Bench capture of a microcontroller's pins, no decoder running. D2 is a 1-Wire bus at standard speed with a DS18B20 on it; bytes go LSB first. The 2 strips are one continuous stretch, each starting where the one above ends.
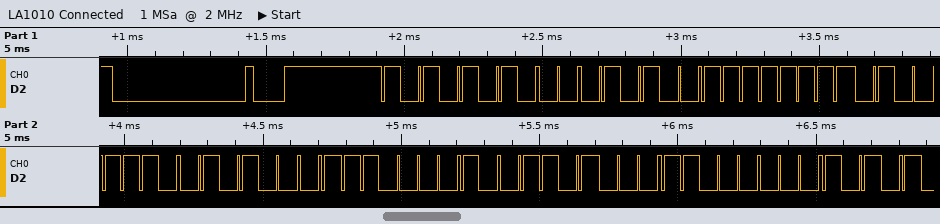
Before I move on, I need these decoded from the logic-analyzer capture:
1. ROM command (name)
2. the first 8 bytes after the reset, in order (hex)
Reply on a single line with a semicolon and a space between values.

Match ROM; 55 28 FF 72 8A 43 16 03
